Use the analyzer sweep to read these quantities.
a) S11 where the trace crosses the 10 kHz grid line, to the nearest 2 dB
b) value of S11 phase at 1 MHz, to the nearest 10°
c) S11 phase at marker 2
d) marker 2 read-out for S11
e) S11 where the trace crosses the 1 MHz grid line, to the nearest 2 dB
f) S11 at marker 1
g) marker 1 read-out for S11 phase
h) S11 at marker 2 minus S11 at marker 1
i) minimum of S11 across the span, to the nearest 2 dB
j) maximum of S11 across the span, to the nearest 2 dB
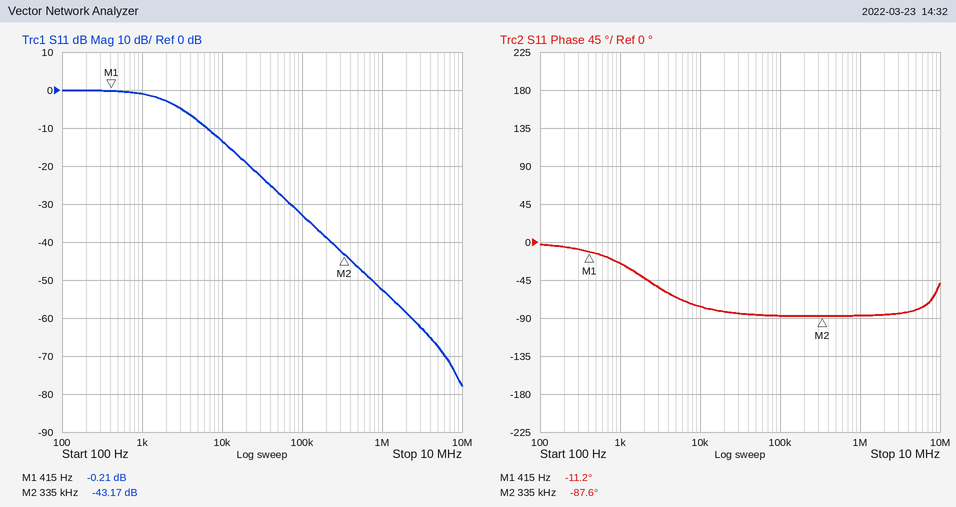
-14 dB
-90°
-87.6°
-43.17 dB
-52 dB
-0.21 dB
-11.2°
-42.96 dB
-78 dB
0 dB
